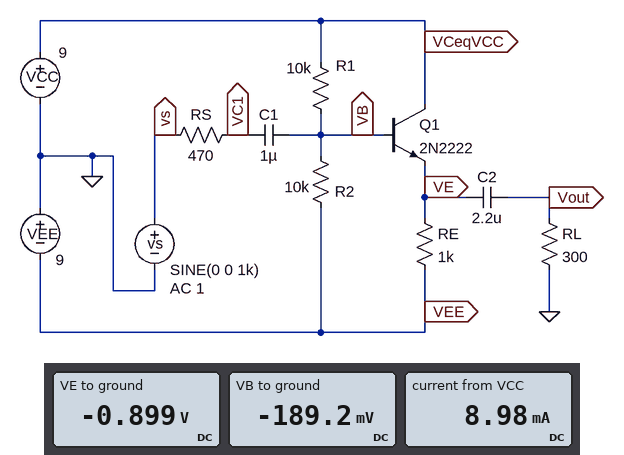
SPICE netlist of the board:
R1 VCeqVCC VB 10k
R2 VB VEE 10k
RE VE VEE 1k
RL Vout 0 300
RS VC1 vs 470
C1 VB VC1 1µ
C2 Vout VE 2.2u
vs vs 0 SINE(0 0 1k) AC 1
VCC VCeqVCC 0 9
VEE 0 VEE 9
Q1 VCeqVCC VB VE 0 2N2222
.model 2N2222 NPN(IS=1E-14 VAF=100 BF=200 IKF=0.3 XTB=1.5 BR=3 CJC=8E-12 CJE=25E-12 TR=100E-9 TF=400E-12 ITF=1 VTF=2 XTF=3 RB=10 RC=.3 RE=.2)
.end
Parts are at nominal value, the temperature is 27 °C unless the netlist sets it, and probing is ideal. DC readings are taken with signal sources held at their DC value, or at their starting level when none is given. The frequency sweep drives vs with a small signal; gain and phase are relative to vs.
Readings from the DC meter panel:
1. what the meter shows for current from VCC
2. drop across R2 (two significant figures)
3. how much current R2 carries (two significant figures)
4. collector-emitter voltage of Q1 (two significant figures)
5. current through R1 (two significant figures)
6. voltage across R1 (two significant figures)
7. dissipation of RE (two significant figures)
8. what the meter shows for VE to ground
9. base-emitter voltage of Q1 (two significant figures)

8.98 mA
8.8 V
880 µA
9.9 V
920 µA
9.2 V
66 mW
-0.899 V
710 mV
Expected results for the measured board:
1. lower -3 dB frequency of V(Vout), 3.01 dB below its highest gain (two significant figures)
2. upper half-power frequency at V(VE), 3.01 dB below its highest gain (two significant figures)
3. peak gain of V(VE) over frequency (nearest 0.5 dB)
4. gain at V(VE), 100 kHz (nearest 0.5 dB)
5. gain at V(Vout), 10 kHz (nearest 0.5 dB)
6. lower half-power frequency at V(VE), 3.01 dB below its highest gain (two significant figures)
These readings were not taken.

240 Hz
60 MHz
-1.0 dB
-1.0 dB
-1.0 dB
29 Hz
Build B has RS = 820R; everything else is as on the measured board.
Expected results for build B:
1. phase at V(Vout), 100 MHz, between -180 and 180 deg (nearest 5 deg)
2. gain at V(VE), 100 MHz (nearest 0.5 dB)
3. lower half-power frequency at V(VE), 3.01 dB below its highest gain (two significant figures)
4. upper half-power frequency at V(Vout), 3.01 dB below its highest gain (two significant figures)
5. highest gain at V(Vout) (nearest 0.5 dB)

-60 deg
-10.5 dB
27 Hz
38 MHz
-1.5 dB
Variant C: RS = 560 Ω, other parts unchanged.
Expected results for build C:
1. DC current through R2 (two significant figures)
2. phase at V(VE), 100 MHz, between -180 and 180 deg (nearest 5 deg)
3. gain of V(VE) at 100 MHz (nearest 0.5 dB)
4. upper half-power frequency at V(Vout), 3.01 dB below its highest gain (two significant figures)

880 µA
-55 deg
-7.5 dB
52 MHz
